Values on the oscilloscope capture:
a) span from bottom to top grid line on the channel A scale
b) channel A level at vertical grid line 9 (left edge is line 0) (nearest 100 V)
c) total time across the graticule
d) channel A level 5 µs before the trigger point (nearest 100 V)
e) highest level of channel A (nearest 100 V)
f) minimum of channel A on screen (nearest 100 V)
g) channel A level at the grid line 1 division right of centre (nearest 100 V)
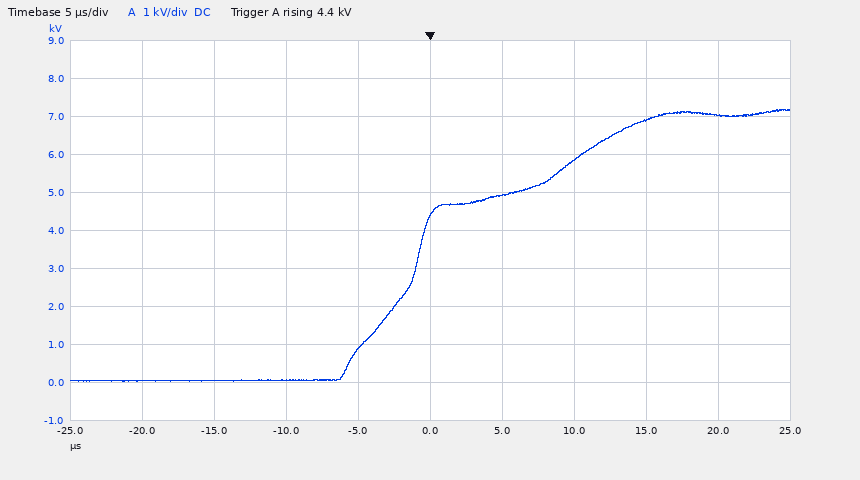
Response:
10 kV
7.0 kV
50 µs
900 V
7.2 kV
0.0 kV
4.9 kV
